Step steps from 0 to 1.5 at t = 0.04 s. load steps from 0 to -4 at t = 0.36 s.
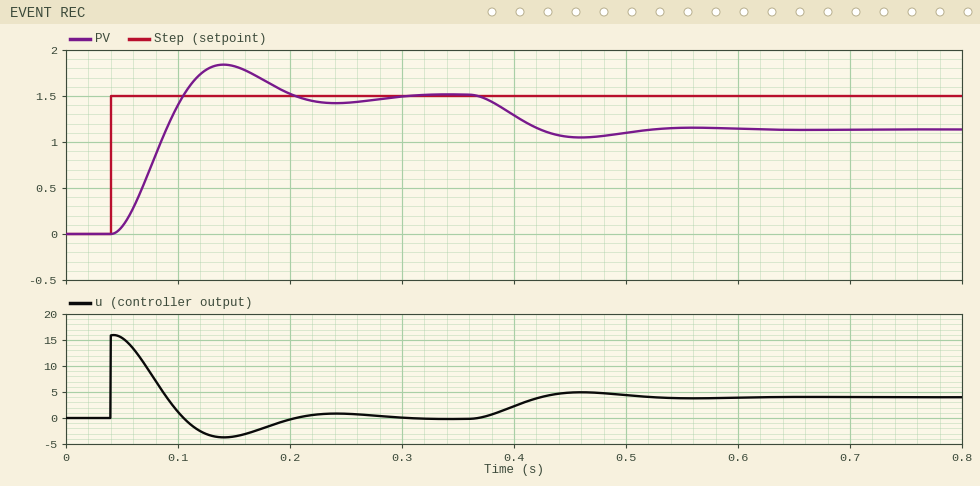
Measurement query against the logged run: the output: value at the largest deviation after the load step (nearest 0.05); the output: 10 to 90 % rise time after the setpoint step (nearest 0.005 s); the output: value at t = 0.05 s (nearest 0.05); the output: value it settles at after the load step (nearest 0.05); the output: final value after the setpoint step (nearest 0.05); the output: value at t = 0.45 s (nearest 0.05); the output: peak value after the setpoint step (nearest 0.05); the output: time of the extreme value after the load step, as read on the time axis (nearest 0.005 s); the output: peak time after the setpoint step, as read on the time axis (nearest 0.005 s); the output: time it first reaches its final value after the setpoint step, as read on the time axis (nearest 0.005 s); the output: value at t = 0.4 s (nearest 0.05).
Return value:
1.05
0.045 s
0.10
1.15
1.50
1.05
1.85
0.460 s
0.140 s
0.105 s
1.30
